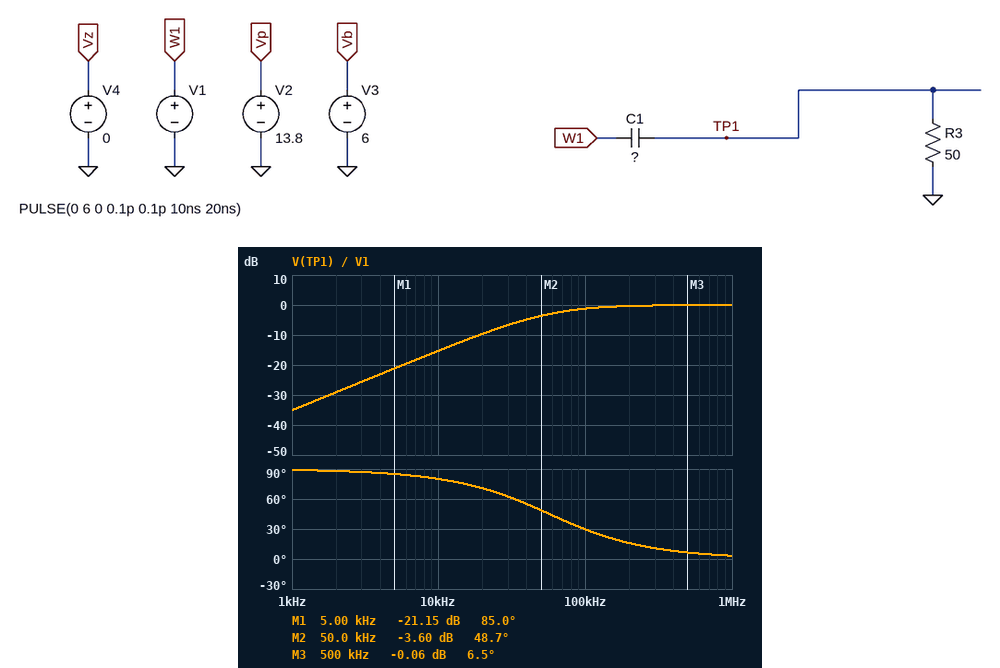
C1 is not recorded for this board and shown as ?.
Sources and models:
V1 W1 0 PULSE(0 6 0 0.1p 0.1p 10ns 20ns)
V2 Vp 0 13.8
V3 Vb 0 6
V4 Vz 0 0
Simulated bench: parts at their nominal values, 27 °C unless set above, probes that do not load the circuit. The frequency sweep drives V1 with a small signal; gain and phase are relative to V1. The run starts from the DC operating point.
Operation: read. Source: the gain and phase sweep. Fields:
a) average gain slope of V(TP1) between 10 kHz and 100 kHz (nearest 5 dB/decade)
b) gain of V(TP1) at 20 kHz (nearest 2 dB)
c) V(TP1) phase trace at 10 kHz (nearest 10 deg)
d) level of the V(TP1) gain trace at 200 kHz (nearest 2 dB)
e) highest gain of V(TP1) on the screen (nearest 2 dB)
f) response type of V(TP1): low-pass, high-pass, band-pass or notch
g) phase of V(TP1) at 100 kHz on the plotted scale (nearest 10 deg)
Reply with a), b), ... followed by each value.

a) 15 dB/decade
b) -10 dB
c) 80 deg
d) 0 dB
e) 0 dB
f) high-pass
g) 30 deg
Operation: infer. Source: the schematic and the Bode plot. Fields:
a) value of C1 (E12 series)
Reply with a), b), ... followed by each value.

a) 56 nF
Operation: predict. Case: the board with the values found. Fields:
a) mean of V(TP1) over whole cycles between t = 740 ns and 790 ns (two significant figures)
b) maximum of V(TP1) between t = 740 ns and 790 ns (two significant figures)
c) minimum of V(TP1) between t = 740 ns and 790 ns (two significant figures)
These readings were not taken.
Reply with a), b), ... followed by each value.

a) 2.3 V
b) 5.3 V
c) -750 mV
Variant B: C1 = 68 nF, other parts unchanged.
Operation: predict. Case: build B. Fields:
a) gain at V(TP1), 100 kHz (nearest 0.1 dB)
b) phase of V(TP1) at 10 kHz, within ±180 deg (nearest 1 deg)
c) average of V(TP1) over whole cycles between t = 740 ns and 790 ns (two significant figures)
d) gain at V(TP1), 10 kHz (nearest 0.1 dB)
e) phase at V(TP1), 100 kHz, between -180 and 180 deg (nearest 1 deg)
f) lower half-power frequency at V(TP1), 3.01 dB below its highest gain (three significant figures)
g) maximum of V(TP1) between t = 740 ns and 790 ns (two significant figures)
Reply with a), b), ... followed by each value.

a) -0.9 dB
b) 78 deg
c) 2.4 V
d) -13.6 dB
e) 25 deg
f) 46.8 kHz
g) 5.4 V
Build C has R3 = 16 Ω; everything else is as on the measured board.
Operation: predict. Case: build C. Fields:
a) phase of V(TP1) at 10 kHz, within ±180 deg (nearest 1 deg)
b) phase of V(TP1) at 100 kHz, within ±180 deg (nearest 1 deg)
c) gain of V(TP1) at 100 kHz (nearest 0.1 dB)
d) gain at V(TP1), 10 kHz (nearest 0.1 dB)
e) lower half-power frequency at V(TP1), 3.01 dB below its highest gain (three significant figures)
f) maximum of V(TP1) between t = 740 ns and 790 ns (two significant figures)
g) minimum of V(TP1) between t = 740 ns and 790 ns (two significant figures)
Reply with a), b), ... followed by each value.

a) 87 deg
b) 61 deg
c) -6.2 dB
d) -25.0 dB
e) 178 kHz
f) 4.3 V
g) -1.8 V
